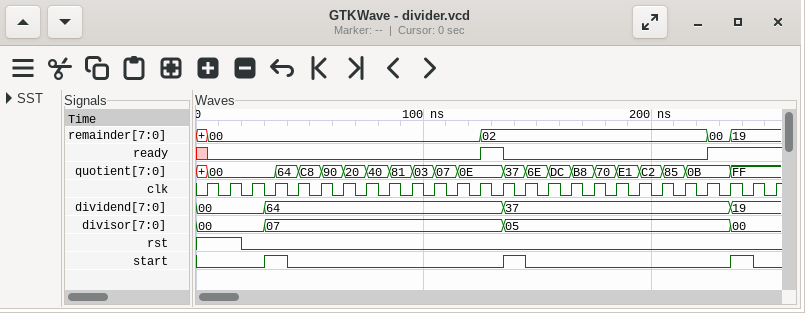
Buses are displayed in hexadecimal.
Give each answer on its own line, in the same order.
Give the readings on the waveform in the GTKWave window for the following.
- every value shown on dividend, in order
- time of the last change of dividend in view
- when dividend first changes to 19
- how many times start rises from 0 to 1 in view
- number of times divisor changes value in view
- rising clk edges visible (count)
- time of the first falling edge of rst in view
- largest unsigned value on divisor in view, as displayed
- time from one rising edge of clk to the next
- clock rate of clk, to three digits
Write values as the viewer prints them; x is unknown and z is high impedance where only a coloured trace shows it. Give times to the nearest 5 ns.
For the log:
00, 64, 37, 19
235 ns
235 ns
3
3
26
20 ns
07
10 ns
100 MHz
